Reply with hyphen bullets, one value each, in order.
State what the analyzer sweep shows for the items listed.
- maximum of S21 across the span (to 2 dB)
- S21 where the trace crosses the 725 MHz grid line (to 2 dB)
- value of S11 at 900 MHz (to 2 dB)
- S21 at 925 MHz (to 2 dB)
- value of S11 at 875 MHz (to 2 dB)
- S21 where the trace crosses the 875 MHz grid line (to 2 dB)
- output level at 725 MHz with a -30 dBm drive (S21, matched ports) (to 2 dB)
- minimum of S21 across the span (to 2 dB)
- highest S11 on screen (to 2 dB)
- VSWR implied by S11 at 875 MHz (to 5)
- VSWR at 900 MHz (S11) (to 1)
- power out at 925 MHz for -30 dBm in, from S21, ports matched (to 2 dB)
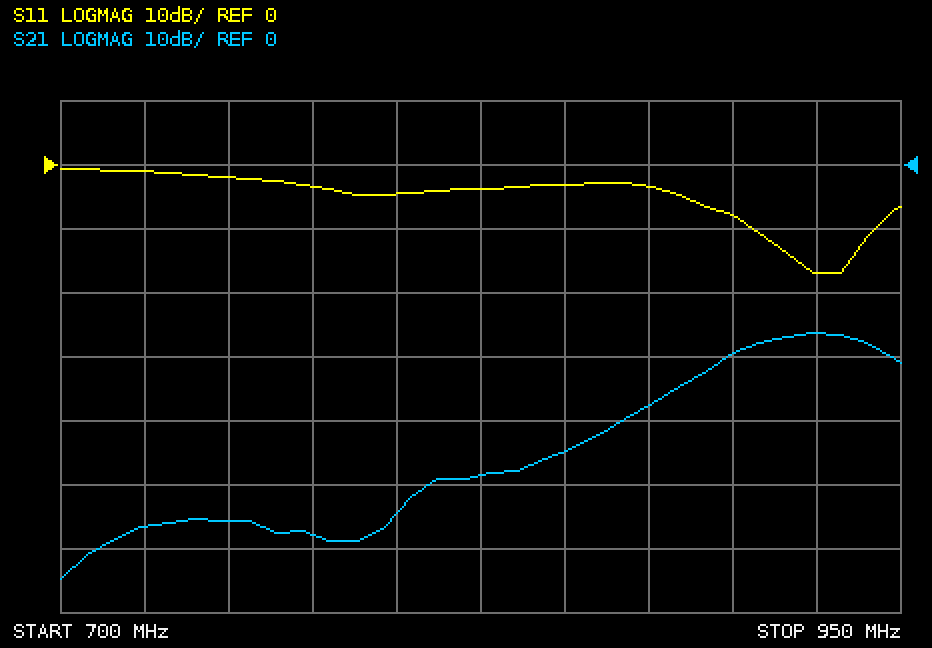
- -26 dB
- -56 dB
- -8 dB
- -26 dB
- -4 dB
- -38 dB
- -86 dBm
- -64 dB
- 0 dB
- 5
- 2
- -56 dBm
